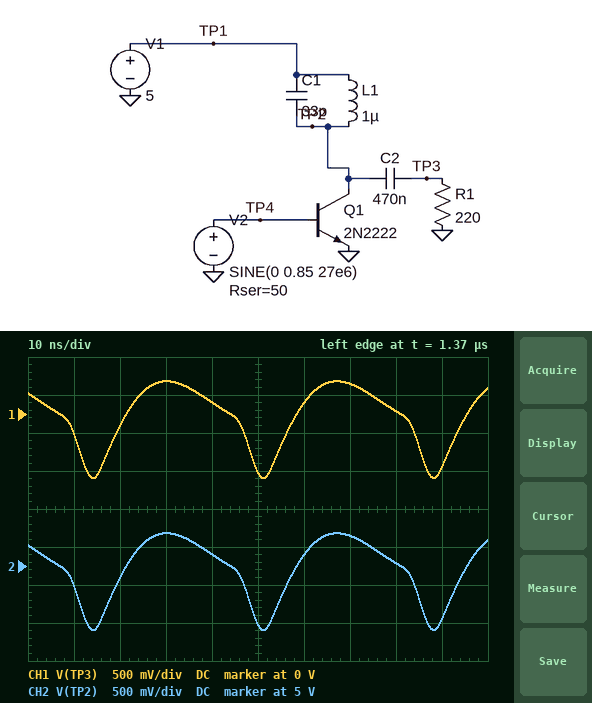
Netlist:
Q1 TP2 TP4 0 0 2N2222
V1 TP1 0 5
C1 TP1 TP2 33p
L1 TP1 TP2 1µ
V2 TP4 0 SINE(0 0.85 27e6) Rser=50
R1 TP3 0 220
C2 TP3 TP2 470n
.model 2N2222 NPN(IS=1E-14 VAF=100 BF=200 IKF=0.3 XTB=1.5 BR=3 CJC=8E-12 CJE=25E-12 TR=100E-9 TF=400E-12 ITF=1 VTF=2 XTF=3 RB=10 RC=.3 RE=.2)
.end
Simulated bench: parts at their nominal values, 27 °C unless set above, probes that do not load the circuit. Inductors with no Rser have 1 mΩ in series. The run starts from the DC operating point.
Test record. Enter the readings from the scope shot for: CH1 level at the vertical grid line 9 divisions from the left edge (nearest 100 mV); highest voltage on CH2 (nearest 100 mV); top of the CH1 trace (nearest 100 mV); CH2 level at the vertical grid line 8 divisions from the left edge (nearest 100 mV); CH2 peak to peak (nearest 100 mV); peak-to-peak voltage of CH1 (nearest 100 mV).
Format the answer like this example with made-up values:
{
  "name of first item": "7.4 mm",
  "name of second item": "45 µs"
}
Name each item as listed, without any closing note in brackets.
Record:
{
  "CH1 level at the vertical grid line 9 divisions from the left edge": "-700 mV",
  "highest voltage on CH2": "5.4 V",
  "top of the CH1 trace": "400 mV",
  "CH2 level at the vertical grid line 8 divisions from the left edge": "5.0 V",
  "CH2 peak to peak": "1.3 V",
  "peak-to-peak voltage of CH1": "1.3 V"
}
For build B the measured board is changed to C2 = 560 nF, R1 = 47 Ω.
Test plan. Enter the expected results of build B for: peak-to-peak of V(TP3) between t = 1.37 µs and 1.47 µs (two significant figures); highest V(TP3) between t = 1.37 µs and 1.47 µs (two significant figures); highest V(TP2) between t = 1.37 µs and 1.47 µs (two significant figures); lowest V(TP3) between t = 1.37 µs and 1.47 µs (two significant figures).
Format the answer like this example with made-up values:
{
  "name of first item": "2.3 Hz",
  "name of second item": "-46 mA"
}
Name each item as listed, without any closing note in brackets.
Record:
{
  "peak-to-peak of V(TP3) between t = 1.37 µs and 1.47 µs": "460 mV",
  "highest V(TP3) between t = 1.37 µs and 1.47 µs": "81 mV",
  "highest V(TP2) between t = 1.37 µs and 1.47 µs": "5.1 V",
  "lowest V(TP3) between t = 1.37 µs and 1.47 µs": "-380 mV"
}
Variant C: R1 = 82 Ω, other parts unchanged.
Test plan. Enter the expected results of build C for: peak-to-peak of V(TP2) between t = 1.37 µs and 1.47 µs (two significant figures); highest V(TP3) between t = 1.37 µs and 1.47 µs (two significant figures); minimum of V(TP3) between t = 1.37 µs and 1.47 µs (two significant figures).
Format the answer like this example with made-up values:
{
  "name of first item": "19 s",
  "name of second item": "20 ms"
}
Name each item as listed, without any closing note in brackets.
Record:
{
  "peak-to-peak of V(TP2) between t = 1.37 µs and 1.47 µs": "680 mV",
  "highest V(TP3) between t = 1.37 µs and 1.47 µs": "150 mV",
  "minimum of V(TP3) between t = 1.37 µs and 1.47 µs": "-530 mV"
}
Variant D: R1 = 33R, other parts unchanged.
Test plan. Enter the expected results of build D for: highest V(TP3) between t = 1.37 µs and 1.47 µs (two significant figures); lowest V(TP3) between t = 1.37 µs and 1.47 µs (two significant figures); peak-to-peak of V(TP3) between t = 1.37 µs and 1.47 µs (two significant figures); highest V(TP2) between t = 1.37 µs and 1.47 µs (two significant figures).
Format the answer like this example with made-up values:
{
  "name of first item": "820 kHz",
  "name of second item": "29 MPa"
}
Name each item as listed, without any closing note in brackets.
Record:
{
  "highest V(TP3) between t = 1.37 µs and 1.47 µs": "60 mV",
  "lowest V(TP3) between t = 1.37 µs and 1.47 µs": "-300 mV",
  "peak-to-peak of V(TP3) between t = 1.37 µs and 1.47 µs": "360 mV",
  "highest V(TP2) between t = 1.37 µs and 1.47 µs": "5.1 V"
}
